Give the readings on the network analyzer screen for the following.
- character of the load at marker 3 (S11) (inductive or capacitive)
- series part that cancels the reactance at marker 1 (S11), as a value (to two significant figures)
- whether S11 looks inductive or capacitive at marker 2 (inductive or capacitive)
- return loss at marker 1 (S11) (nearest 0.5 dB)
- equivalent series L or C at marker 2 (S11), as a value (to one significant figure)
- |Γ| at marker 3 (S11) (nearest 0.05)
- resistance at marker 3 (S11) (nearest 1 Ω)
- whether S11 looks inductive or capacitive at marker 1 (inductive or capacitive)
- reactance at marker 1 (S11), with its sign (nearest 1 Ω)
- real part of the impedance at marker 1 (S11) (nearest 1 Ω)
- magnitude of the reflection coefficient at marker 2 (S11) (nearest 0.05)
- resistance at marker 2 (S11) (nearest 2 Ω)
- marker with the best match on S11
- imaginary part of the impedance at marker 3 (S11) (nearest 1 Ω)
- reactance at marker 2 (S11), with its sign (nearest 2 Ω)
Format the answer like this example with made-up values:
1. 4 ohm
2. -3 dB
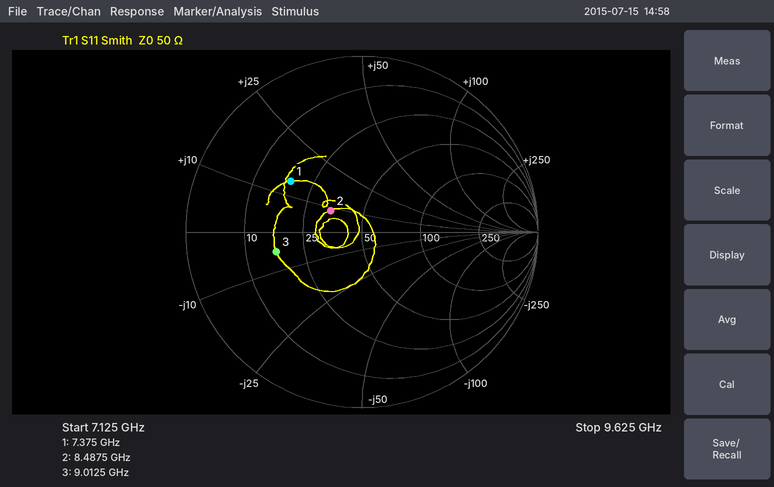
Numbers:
1. capacitive
2. 1.5 pF
3. inductive
4. 6.0 dB
5. 200 pH
6. 0.50
7. 17 Ω
8. inductive
9. +14 Ω
10. 18 Ω
11. 0.20
12. 34 Ω
13. marker 2
14. -5 Ω
15. +8 Ω
